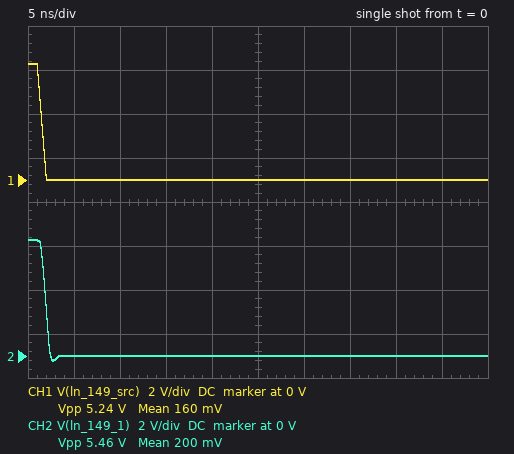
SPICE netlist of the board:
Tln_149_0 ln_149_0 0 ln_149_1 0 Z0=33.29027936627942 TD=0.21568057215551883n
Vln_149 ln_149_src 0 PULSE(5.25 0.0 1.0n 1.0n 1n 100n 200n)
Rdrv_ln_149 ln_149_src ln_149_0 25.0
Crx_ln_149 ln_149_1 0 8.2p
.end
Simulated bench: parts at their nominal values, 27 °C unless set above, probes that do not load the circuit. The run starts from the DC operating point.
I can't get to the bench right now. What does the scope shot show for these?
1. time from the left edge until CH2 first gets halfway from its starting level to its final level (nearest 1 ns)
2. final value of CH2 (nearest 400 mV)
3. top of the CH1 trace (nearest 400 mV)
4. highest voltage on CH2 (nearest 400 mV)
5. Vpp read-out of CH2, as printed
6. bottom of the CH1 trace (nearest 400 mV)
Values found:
2 ns
0 V
5.2 V
5.2 V
5.46 V
0 V
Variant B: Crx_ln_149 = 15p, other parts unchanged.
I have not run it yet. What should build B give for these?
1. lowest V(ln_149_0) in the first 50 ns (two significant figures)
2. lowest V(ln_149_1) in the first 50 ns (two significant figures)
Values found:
-50 mV
-79 mV
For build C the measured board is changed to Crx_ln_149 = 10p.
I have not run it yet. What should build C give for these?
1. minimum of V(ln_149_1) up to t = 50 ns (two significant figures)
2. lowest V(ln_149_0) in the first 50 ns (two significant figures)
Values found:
-180 mV
-100 mV
